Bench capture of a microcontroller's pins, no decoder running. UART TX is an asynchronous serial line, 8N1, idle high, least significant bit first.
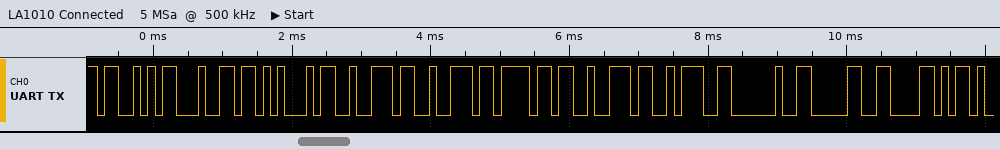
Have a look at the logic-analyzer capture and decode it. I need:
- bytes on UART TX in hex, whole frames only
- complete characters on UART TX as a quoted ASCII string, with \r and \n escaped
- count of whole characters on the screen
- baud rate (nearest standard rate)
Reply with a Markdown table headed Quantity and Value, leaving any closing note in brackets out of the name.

| Quantity | Value |
|---|---|
| bytes on UART TX in hex, whole frames only | 0x53 0x64 0x45 0x72 0x72 0x6F 0x72 0x3A 0x20 0x30 0x58 |
| complete characters on UART TX as a quoted ASCII string, with \r and \n escaped | "SdError: 0X" |
| count of whole characters on the screen | 11 |
| baud rate | 9600 baud |
